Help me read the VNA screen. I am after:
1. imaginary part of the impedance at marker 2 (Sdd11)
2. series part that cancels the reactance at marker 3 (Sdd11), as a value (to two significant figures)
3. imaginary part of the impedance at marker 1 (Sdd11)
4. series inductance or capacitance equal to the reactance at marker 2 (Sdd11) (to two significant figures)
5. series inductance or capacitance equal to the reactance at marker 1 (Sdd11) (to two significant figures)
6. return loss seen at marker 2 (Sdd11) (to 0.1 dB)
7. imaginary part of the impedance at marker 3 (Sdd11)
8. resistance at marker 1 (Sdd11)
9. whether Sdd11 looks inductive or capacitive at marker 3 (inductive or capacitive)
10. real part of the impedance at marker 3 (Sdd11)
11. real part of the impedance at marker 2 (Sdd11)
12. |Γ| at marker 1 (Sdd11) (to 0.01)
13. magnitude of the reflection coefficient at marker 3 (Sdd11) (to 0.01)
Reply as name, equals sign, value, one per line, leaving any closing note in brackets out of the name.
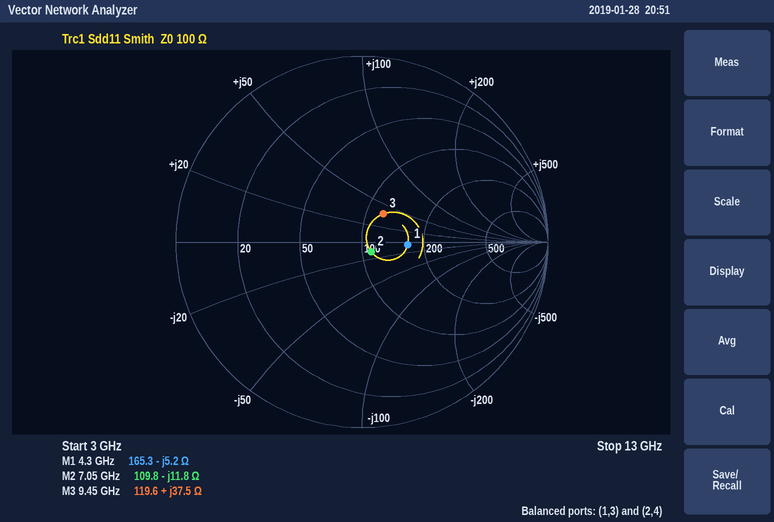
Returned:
imaginary part of the impedance at marker 2 = -11.8 Ω
series part that cancels the reactance at marker 3 (Sdd11), as a value = 450 fF
imaginary part of the impedance at marker 1 = -5.2 Ω
series inductance or capacitance equal to the reactance at marker 2 (Sdd11) = 1.9 pF
series inductance or capacitance equal to the reactance at marker 1 (Sdd11) = 7.1 pF
return loss seen at marker 2 (Sdd11) = 22.7 dB
imaginary part of the impedance at marker 3 = +37.5 Ω
resistance at marker 1 = 165.3 Ω
whether Sdd11 looks inductive or capacitive at marker 3 = inductive
real part of the impedance at marker 3 = 119.6 Ω
real part of the impedance at marker 2 = 109.8 Ω
|Γ| at marker 1 (Sdd11) = 0.25
magnitude of the reflection coefficient at marker 3 (Sdd11) = 0.19
